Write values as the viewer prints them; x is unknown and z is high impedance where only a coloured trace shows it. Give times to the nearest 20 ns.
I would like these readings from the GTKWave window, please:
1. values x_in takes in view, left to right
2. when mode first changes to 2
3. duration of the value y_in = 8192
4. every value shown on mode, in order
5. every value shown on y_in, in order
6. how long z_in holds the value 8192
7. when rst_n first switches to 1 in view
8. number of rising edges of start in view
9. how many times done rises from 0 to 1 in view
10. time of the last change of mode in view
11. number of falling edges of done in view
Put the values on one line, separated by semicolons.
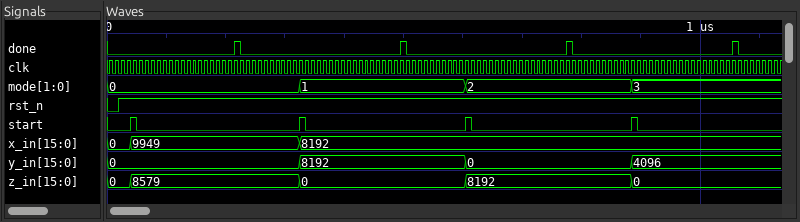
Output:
0, 9949, 8192; 600 ns; 280 ns; 0, 1, 2, 3; 0, 8192, 0, 4096; 280 ns; 20 ns; 4; 4; 880 ns; 4
